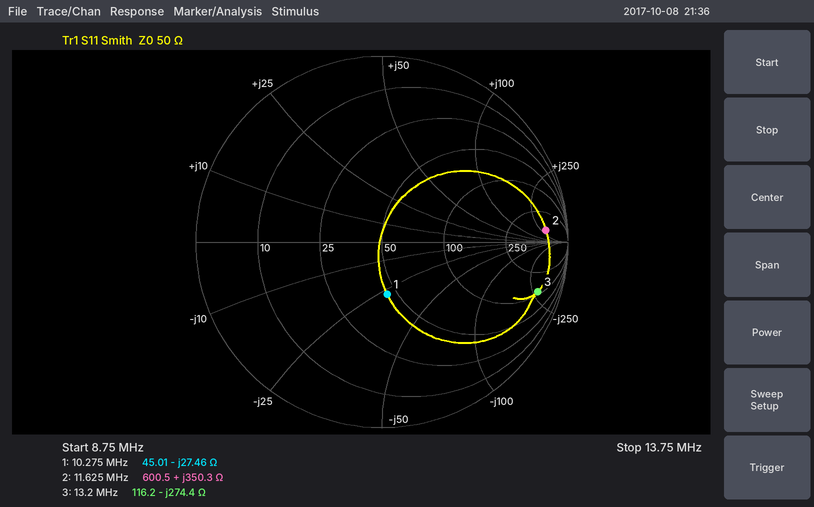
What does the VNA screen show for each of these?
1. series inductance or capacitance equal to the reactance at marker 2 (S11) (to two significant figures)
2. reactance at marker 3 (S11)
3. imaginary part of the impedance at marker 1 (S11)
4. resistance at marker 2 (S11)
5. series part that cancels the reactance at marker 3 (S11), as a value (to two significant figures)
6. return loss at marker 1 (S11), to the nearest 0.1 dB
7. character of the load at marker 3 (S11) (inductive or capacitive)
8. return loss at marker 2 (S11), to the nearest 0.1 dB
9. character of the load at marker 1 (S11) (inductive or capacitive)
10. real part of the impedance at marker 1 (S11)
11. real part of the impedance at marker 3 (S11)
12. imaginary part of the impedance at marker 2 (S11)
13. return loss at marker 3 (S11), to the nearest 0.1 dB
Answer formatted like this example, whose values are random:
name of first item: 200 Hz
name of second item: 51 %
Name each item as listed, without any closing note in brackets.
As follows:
series inductance or capacitance equal to the reactance at marker 2 (S11): 4.8 µH
reactance at marker 3: -274.4 Ω
imaginary part of the impedance at marker 1: -27.46 Ω
resistance at marker 2: 600.5 Ω
series part that cancels the reactance at marker 3 (S11), as a value: 3.3 µH
return loss at marker 1 (S11), to the nearest 0.1 dB: 11.0 dB
character of the load at marker 3 (S11): capacitive
return loss at marker 2 (S11), to the nearest 0.1 dB: 1.1 dB
character of the load at marker 1 (S11): capacitive
real part of the impedance at marker 1: 45.01 Ω
real part of the impedance at marker 3: 116.2 Ω
imaginary part of the impedance at marker 2: +350.3 Ω
return loss at marker 3 (S11), to the nearest 0.1 dB: 1.1 dB
